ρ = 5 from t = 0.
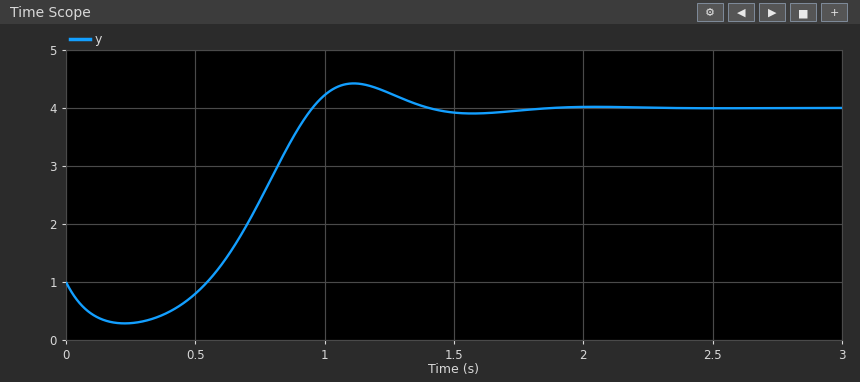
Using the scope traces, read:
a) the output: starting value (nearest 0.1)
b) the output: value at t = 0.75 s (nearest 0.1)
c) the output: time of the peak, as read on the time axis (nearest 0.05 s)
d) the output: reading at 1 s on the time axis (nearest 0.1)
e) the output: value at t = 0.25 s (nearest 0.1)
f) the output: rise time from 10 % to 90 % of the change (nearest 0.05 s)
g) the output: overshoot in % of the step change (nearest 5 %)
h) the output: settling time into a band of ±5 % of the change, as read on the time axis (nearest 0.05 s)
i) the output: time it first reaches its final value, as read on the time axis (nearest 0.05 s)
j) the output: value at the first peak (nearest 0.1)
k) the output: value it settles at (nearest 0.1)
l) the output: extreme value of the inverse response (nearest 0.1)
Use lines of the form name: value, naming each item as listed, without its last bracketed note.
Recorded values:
the output: starting value: 1.0
the output: value at t = 0.75 s: 2.4
the output: time of the peak, as read on the time axis: 1.10 s
the output: reading at 1 s on the time axis: 4.2
the output: value at t = 0.25 s: 0.3
the output: rise time from 10 % to 90 % of the change: 0.30 s
the output: overshoot in % of the step change: 15 %
the output: settling time into a band of ±5 % of the change, as read on the time axis: 1.30 s
the output: time it first reaches its final value, as read on the time axis: 0.95 s
the output: value at the first peak: 4.4
the output: value it settles at: 4.0
the output: extreme value of the inverse response: 0.3
